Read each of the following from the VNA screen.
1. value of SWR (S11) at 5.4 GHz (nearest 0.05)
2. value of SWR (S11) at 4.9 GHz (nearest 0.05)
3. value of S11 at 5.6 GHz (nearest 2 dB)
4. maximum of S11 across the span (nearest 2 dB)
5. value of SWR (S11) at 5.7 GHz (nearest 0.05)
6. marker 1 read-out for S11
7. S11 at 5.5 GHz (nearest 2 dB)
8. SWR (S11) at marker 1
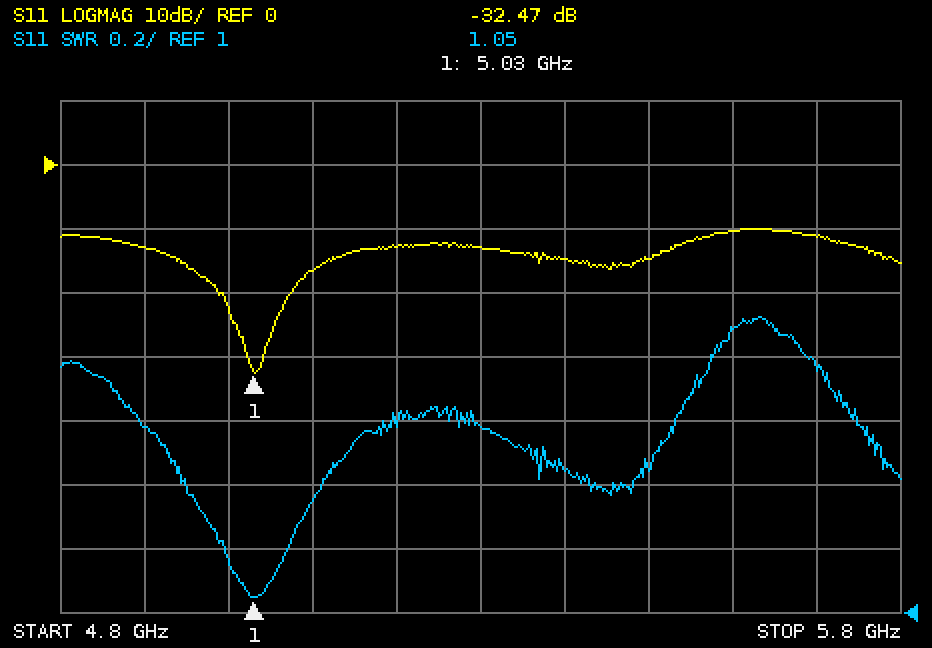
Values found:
1.45
1.60
-10 dB
-10 dB
1.75
-32.47 dB
-14 dB
1.05
